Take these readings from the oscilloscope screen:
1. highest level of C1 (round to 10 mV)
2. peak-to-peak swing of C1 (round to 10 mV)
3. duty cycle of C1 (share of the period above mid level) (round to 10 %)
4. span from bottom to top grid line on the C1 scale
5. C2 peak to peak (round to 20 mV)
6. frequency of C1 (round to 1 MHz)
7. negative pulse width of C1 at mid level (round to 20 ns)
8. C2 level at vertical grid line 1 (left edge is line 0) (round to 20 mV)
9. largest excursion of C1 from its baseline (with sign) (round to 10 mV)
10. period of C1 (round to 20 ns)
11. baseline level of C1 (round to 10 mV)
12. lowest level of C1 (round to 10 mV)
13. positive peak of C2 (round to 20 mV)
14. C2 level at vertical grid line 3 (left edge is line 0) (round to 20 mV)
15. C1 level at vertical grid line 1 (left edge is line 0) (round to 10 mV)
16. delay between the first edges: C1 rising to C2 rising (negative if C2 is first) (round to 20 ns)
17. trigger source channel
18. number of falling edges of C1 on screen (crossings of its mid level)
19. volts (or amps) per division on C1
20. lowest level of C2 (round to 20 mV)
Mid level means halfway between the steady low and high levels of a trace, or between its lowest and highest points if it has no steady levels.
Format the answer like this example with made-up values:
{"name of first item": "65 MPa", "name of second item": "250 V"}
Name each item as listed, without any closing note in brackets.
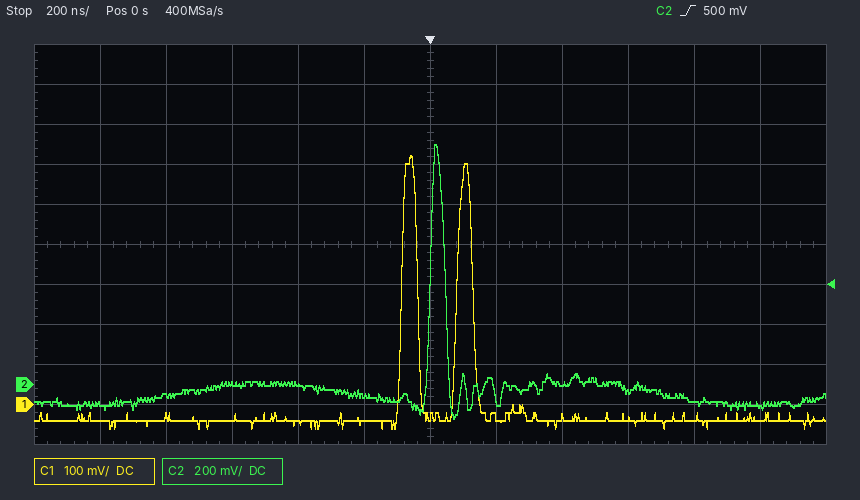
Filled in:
{"highest level of C1": "620 mV", "peak-to-peak swing of C1": "680 mV", "duty cycle of C1 (share of the period above mid level)": "30 %", "span from bottom to top grid line on the C1 scale": "1 V", "C2 peak to peak": "1.36 V", "frequency of C1": "6 MHz", "negative pulse width of C1 at mid level": "120 ns", "C2 level at vertical grid line 1 (left edge is line 0)": "-100 mV", "largest excursion of C1 from its baseline (with sign)": "+660 mV", "period of C1": "160 ns", "baseline level of C1": "-40 mV", "lowest level of C1": "-60 mV", "positive peak of C2": "1.20 V", "C2 level at vertical grid line 3 (left edge is line 0)": "0 mV", "C1 level at vertical grid line 1 (left edge is line 0)": "-40 mV", "delay between the first edges: C1 rising to C2 rising (negative if C2 is first)": "+80 ns", "trigger source channel": "C2", "number of falling edges of C1 on screen": "2", "volts (or amps) per division on C1": "100 mV", "lowest level of C2": "-160 mV"}
